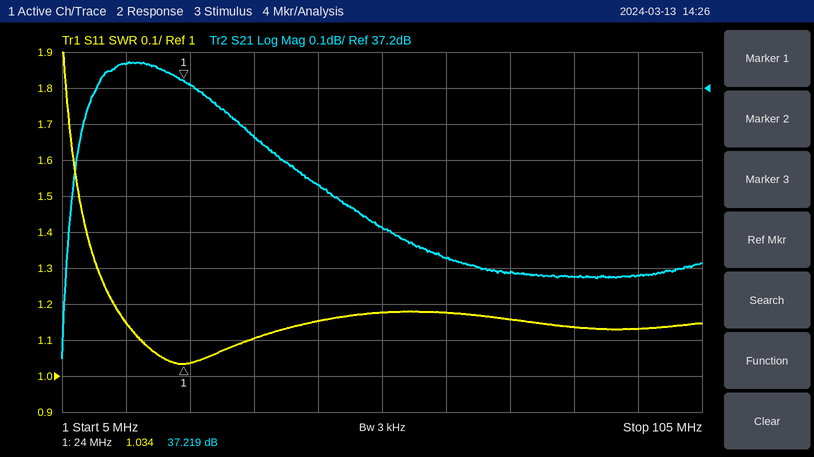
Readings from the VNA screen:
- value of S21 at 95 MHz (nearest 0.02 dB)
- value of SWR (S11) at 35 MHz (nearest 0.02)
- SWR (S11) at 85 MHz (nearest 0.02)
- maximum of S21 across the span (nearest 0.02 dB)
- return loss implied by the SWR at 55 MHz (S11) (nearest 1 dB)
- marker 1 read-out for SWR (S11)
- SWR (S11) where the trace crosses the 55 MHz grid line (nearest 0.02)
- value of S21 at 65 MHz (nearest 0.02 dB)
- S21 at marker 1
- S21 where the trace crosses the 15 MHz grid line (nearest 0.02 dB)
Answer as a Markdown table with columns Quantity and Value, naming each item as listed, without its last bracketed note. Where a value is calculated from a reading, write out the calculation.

| Quantity | Value |
|---|---|
| value of S21 at 95 MHz | 36.68 dB |
| value of SWR (S11) at 35 MHz | 1.10 |
| SWR (S11) at 85 MHz | 1.14 |
| maximum of S21 across the span | 37.28 dB |
| return loss implied by the SWR at 55 MHz (S11) | −20 log10((1.18 − 1)/(1.18 + 1)) ≈ 22 dB |
| marker 1 read-out for SWR | 1.034 |
| SWR (S11) where the trace crosses the 55 MHz grid line | 1.18 |
| value of S21 at 65 MHz | 36.72 dB |
| S21 at marker 1 | 37.219 dB |
| S21 where the trace crosses the 15 MHz grid line | 37.26 dB |
